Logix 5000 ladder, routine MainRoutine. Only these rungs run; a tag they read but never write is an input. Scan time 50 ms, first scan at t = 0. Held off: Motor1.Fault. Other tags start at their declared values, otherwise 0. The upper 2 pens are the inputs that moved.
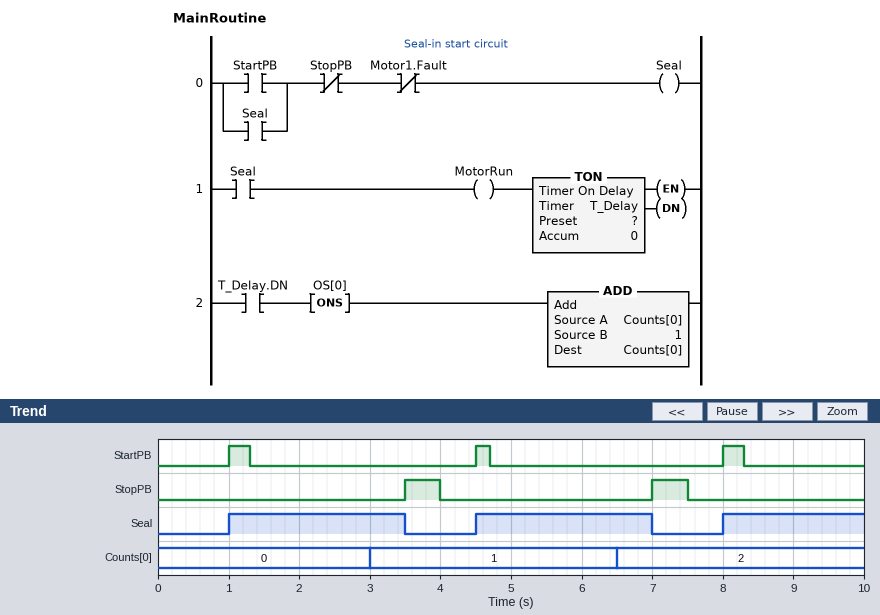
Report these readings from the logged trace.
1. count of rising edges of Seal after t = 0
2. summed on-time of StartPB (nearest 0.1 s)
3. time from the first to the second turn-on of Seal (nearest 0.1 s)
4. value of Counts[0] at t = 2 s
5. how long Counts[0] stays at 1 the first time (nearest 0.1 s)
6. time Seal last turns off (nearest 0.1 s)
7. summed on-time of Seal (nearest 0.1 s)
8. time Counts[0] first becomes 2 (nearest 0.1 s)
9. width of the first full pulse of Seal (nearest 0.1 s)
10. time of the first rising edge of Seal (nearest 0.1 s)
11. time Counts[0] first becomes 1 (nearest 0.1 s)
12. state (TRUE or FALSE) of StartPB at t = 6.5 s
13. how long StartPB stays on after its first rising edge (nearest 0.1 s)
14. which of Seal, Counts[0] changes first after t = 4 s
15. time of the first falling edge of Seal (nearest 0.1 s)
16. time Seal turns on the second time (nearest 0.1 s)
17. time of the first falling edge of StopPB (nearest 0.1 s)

3
0.8 s
3.5 s
0
3.5 s
7.0 s
7.0 s
6.5 s
2.5 s
1.0 s
3.0 s
FALSE
0.3 s
Seal
3.5 s
4.5 s
4.0 s
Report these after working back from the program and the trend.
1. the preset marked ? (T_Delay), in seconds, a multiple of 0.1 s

2.0 s
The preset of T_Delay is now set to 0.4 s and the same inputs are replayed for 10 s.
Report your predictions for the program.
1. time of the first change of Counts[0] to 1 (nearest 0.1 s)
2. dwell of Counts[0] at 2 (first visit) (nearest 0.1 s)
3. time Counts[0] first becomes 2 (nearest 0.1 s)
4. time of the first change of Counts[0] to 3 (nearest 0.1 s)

1.4 s
3.5 s
4.9 s
8.4 s
